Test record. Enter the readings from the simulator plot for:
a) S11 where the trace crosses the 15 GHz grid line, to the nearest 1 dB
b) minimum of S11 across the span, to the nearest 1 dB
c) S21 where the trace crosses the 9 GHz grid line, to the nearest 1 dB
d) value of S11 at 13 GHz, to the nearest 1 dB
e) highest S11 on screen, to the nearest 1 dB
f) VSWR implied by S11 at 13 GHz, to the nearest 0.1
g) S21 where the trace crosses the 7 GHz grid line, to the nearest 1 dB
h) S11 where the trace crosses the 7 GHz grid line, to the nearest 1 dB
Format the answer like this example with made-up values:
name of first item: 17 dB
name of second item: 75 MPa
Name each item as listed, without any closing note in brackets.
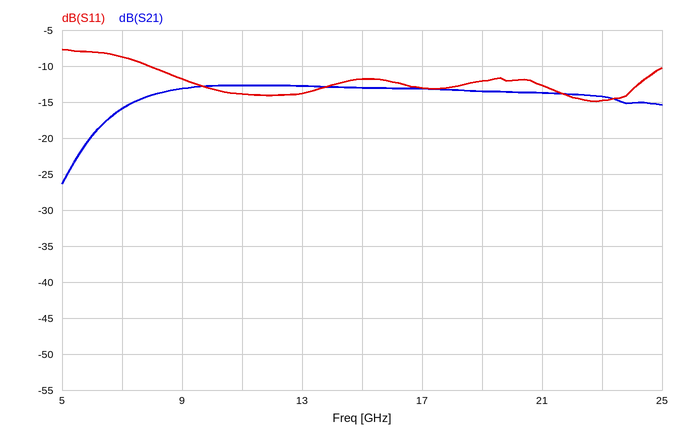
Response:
S11 where the trace crosses the 15 GHz grid line, to the nearest 1 dB: -12 dB
minimum of S11 across the span, to the nearest 1 dB: -15 dB
S21 where the trace crosses the 9 GHz grid line, to the nearest 1 dB: -13 dB
value of S11 at 13 GHz, to the nearest 1 dB: -14 dB
highest S11 on screen, to the nearest 1 dB: -8 dB
VSWR implied by S11 at 13 GHz, to the nearest 0.1: 1.5
S21 where the trace crosses the 7 GHz grid line, to the nearest 1 dB: -16 dB
S11 where the trace crosses the 7 GHz grid line, to the nearest 1 dB: -9 dB
